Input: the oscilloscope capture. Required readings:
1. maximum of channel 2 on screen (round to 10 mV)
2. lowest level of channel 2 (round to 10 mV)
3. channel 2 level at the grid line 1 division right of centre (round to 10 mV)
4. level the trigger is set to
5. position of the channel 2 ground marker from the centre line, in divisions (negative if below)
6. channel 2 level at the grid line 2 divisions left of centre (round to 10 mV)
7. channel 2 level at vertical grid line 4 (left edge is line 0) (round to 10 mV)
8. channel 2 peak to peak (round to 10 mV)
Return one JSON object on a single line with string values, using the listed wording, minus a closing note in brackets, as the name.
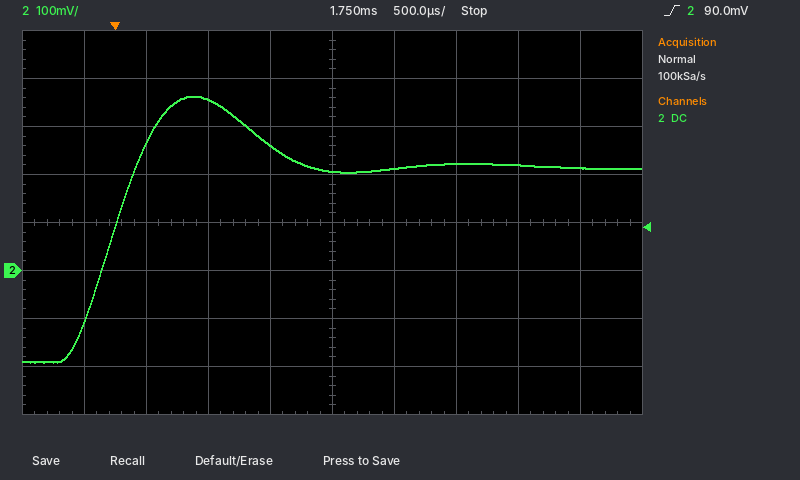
{"maximum of channel 2 on screen": "360 mV", "lowest level of channel 2": "-190 mV", "channel 2 level at the grid line 1 division right of centre": "210 mV", "level the trigger is set to": "90.0 mV", "position of the channel 2 ground marker from the centre line, in divisions": "-1.0 div", "channel 2 level at the grid line 2 divisions left of centre": "360 mV", "channel 2 level at vertical grid line 4 (left edge is line 0)": "260 mV", "channel 2 peak to peak": "550 mV"}
